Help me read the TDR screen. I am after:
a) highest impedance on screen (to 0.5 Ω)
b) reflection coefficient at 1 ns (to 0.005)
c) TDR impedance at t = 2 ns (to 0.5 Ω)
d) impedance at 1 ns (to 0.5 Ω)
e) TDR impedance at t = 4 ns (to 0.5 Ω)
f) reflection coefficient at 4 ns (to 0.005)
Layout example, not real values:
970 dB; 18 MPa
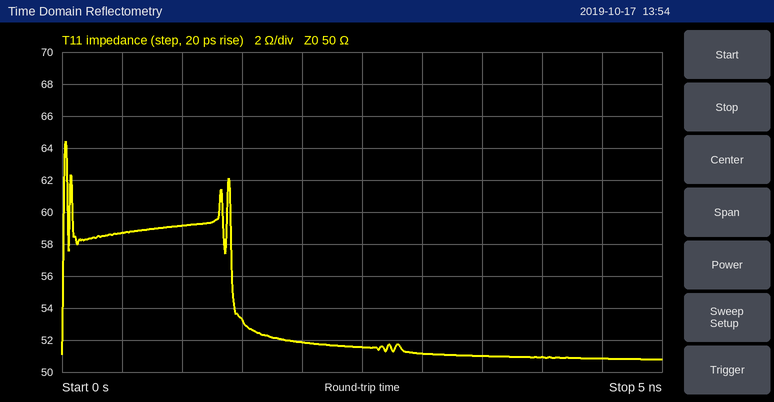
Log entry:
64.5 Ω; +0.085; 52.0 Ω; 59.0 Ω; 51.0 Ω; +0.010
